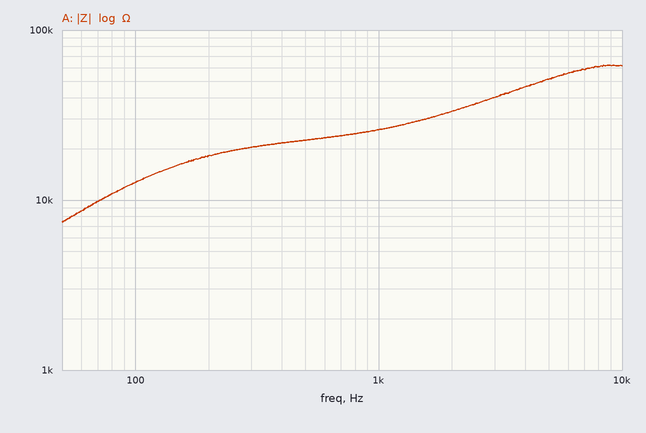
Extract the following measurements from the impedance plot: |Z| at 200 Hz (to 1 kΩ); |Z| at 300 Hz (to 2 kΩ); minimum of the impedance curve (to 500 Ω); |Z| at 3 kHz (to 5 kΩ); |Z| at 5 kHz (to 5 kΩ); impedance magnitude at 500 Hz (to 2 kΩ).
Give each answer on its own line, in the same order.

18 kΩ
20 kΩ
7.5 kΩ
40 kΩ
50 kΩ
22 kΩ
